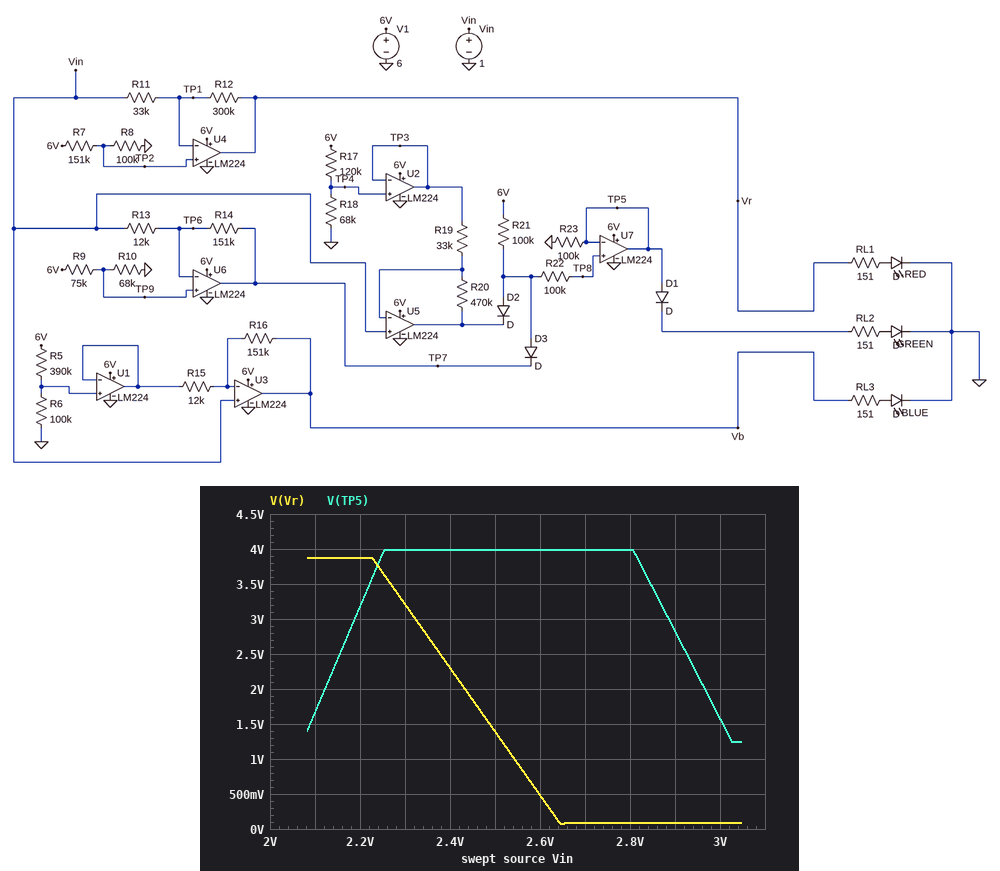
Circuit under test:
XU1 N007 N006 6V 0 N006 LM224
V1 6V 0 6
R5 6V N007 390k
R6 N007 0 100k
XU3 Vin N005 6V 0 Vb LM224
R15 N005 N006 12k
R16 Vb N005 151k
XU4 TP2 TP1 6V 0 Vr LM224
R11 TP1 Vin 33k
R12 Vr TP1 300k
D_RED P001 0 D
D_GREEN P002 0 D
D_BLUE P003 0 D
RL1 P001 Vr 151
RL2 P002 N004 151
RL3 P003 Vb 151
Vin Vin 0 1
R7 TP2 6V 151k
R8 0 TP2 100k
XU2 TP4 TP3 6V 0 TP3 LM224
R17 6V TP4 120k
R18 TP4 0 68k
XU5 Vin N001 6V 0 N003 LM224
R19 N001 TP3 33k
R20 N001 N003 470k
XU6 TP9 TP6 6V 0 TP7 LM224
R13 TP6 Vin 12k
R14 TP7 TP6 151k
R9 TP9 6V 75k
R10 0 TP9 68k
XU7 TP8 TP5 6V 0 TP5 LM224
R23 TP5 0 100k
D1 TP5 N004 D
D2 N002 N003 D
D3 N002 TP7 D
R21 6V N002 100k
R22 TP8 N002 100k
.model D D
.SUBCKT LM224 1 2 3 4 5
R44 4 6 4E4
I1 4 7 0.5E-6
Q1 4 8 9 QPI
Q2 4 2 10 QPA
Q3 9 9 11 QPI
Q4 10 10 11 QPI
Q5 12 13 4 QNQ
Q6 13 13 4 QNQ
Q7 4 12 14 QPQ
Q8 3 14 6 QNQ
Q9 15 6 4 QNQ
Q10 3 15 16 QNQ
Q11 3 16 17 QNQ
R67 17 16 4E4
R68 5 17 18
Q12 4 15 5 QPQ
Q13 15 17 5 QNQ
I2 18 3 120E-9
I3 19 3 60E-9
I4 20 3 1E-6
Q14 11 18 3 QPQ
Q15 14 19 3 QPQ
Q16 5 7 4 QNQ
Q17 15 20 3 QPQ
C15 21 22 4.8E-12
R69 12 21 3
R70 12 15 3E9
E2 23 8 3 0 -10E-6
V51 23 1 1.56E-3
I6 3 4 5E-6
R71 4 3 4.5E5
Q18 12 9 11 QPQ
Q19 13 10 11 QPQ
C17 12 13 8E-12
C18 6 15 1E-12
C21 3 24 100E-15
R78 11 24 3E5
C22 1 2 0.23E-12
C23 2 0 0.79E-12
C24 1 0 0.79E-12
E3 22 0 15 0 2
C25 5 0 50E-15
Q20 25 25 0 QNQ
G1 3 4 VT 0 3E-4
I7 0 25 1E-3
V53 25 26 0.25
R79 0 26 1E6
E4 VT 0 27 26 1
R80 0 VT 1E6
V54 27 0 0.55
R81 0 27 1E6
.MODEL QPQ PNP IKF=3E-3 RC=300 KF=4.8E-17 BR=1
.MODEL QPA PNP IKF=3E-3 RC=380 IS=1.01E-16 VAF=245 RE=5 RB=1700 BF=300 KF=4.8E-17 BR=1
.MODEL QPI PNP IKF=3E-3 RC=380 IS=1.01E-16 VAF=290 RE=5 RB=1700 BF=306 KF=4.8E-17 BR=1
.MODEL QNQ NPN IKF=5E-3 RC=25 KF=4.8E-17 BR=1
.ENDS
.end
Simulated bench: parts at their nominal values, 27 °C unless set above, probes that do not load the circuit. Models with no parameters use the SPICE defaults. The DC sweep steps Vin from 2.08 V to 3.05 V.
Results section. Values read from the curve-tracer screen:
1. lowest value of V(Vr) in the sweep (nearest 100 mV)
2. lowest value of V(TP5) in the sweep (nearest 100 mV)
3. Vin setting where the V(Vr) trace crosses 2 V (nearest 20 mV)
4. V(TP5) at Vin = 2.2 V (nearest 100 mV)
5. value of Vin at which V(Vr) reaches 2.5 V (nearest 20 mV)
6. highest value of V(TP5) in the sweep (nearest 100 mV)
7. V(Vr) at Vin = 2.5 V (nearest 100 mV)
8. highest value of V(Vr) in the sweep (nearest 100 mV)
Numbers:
100 mV
1.2 V
2.44 V
3.2 V
2.38 V
4.0 V
1.4 V
3.9 V
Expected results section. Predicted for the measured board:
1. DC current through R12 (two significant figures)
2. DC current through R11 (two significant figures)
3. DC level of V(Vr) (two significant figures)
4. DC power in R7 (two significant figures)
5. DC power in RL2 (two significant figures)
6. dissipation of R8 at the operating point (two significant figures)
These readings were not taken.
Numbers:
8.6 µA
8.7 µA
3.9 V
86 µW
770 nW
57 µW
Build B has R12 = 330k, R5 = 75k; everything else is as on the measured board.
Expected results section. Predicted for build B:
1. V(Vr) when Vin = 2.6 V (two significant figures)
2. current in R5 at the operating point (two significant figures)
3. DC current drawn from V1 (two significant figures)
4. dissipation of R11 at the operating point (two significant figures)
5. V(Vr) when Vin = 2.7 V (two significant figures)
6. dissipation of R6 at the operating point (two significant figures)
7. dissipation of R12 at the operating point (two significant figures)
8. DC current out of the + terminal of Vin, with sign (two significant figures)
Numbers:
290 mV
34 µA
23 mA
2.1 µW
77 mV
120 µW
21 µW
-30 µA
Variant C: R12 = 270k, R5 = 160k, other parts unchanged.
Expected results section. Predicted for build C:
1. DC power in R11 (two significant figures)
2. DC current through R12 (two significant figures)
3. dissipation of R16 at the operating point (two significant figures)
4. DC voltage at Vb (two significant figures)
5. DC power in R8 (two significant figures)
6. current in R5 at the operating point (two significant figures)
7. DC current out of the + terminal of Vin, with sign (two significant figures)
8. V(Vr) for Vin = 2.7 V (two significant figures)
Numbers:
3.0 µW
9.5 µA
28 µW
96 mV
57 µW
23 µA
-32 µA
82 mV
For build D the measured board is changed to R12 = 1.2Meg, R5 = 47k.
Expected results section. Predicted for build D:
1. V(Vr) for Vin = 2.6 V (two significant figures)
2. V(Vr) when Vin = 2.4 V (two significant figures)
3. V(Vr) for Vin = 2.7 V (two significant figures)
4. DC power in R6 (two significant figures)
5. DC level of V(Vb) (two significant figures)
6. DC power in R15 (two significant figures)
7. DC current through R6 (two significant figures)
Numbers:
48 mV
2.0 V
49 mV
170 µW
120 mV
7.1 µW
41 µA
